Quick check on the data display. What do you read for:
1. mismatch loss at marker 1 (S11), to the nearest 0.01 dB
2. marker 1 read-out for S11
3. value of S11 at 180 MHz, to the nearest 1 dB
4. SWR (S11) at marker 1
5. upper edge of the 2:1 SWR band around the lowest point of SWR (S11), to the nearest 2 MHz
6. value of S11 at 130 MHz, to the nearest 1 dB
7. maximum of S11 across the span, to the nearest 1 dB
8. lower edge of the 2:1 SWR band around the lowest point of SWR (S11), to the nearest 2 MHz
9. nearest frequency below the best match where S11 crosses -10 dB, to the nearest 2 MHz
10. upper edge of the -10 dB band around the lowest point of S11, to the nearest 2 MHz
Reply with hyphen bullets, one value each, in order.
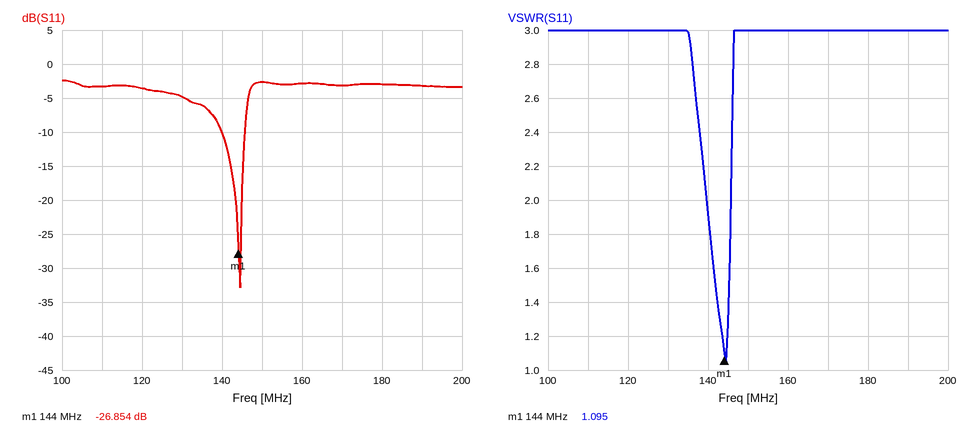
- 0.01 dB
- -26.854 dB
- -3 dB
- 1.095
- 146 MHz
- -5 dB
- -2 dB
- 140 MHz
- 140 MHz
- 146 MHz
